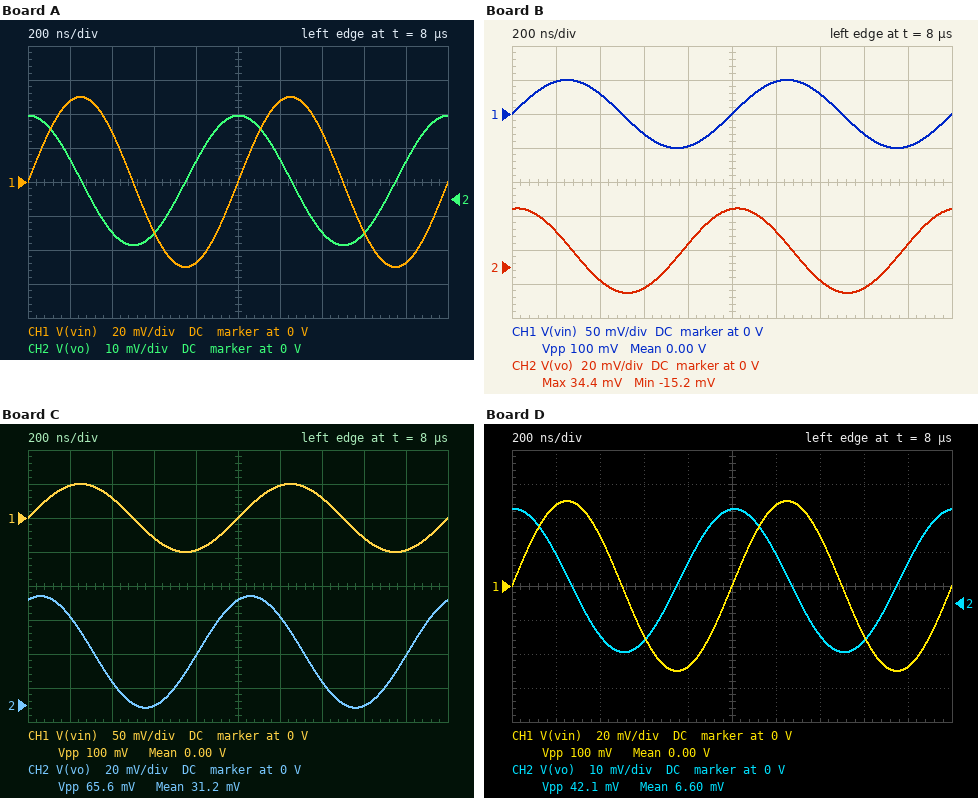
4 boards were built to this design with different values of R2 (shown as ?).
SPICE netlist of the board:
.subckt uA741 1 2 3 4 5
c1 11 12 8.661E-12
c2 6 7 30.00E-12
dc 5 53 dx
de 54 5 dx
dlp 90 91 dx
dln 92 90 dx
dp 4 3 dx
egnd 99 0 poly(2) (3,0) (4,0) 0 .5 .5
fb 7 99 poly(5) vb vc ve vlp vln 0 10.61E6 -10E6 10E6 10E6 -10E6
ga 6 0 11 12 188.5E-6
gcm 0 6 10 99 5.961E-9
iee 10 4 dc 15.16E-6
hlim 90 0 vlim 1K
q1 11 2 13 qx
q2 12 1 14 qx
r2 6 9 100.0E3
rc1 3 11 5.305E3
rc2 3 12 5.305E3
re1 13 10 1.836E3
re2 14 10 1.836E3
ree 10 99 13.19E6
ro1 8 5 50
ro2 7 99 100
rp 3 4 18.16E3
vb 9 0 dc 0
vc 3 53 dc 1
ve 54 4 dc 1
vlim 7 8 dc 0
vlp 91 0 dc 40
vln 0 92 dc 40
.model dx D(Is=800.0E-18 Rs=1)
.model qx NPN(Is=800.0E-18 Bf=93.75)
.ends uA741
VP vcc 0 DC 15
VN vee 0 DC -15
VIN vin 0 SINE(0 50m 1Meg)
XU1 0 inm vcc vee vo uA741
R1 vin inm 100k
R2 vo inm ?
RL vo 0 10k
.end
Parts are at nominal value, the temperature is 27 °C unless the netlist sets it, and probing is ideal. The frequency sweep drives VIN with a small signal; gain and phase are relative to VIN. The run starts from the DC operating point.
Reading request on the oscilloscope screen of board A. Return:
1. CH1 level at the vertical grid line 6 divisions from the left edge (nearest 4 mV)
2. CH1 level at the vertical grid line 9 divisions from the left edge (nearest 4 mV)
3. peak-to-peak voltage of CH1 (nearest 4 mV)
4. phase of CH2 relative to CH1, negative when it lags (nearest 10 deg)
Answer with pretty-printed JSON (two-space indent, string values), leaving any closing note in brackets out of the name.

{
  "CH1 level at the vertical grid line 6 divisions from the left edge": "48 mV",
  "CH1 level at the vertical grid line 9 divisions from the left edge": "-48 mV",
  "peak-to-peak voltage of CH1": "100 mV",
  "phase of CH2 relative to CH1, negative when it lags": "90 deg"
}
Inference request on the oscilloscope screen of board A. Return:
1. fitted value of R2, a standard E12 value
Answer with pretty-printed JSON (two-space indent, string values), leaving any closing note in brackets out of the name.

{
  "fitted value of R2, a standard E12 value": "68 kΩ"
}
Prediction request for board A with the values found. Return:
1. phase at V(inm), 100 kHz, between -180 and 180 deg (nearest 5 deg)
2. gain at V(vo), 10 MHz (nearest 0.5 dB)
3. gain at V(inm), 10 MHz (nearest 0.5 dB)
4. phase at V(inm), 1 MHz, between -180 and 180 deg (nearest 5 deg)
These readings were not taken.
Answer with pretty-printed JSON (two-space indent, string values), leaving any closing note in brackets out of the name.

{
  "phase at V(inm), 100 kHz, between -180 and 180 deg": "85 deg",
  "gain at V(vo), 10 MHz": "-43.0 dB",
  "gain at V(inm), 10 MHz": "-8.0 dB",
  "phase at V(inm), 1 MHz, between -180 and 180 deg": "30 deg"
}
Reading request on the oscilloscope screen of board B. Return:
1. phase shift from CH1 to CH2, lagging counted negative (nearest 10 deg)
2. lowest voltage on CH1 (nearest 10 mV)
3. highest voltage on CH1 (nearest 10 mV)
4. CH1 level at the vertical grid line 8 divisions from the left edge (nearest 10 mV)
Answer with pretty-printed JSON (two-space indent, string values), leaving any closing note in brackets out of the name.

{
  "phase shift from CH1 to CH2, lagging counted negative": "80 deg",
  "lowest voltage on CH1": "-50 mV",
  "highest voltage on CH1": "50 mV",
  "CH1 level at the vertical grid line 8 divisions from the left edge": "-30 mV"
}
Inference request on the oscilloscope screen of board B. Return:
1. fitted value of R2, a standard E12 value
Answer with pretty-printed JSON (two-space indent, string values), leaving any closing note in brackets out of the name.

{
  "fitted value of R2, a standard E12 value": "120 kΩ"
}
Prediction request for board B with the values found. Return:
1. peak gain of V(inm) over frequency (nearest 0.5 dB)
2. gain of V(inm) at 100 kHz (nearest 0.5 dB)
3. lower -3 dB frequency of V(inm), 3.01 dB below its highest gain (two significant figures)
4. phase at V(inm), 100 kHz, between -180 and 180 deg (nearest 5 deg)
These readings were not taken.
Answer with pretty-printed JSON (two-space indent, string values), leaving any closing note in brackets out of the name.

{
  "peak gain of V(inm) over frequency": "-4.5 dB",
  "gain of V(inm) at 100 kHz": "-18.5 dB",
  "lower -3 dB frequency of V(inm), 3.01 dB below its highest gain": "420 kHz",
  "phase at V(inm), 100 kHz, between -180 and 180 deg": "80 deg"
}
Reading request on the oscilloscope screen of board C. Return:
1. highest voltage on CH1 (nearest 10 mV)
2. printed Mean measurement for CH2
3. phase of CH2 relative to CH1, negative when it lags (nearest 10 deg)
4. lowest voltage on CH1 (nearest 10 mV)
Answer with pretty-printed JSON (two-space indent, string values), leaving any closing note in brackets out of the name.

{
  "highest voltage on CH1": "50 mV",
  "printed Mean measurement for CH2": "31.2 mV",
  "phase of CH2 relative to CH1, negative when it lags": "70 deg",
  "lowest voltage on CH1": "-50 mV"
}
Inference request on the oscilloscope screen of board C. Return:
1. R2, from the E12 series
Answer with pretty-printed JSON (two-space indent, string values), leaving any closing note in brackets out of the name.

{
  "R2, from the E12 series": "390 kΩ"
}
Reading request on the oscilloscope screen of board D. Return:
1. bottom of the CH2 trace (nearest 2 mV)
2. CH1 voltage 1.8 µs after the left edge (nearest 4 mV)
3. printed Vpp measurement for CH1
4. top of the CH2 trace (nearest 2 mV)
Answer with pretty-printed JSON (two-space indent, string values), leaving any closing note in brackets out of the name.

{
  "bottom of the CH2 trace": "-14 mV",
  "CH1 voltage 1.8 µs after the left edge": "-48 mV",
  "printed Vpp measurement for CH1": "100 mV",
  "top of the CH2 trace": "28 mV"
}
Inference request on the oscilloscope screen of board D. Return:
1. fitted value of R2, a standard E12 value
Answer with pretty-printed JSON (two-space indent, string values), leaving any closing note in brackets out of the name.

{
  "fitted value of R2, a standard E12 value": "82 kΩ"
}
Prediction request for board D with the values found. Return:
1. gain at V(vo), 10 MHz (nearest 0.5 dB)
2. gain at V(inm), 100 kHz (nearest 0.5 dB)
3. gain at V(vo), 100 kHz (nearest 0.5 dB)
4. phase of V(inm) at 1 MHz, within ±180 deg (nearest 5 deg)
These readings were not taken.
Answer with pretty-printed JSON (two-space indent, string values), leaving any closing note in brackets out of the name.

{
  "gain at V(vo), 10 MHz": "-42.5 dB",
  "gain at V(inm), 100 kHz": "-21.5 dB",
  "gain at V(vo), 100 kHz": "-2.0 dB",
  "phase of V(inm) at 1 MHz, within ±180 deg": "25 deg"
}
